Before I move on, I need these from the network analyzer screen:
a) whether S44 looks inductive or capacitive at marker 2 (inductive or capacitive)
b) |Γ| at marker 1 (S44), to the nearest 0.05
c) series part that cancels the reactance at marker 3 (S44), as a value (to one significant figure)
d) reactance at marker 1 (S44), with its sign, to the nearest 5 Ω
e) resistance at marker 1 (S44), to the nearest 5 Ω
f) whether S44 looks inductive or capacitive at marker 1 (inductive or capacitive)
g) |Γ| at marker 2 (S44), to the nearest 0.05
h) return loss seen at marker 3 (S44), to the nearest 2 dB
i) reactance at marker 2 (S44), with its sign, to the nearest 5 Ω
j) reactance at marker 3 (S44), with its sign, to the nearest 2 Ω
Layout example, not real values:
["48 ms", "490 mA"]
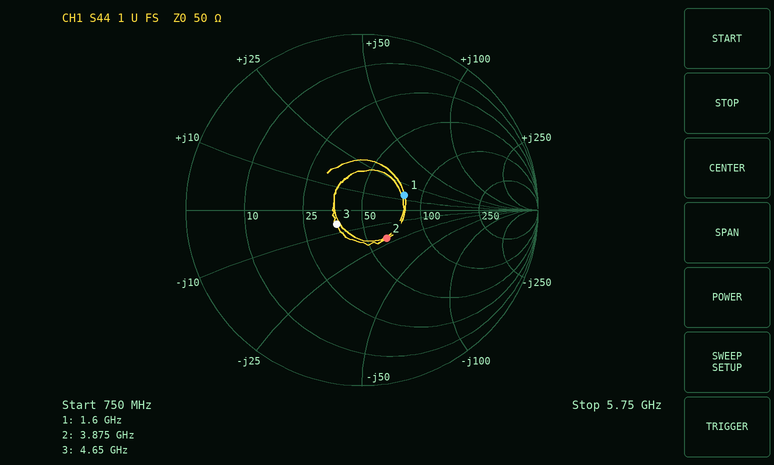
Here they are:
["capacitive", "0.25", "200 pH", "+15 Ω", "80 Ω", "inductive", "0.20", "16 dB", "-20 Ω", "-6 Ω"]
